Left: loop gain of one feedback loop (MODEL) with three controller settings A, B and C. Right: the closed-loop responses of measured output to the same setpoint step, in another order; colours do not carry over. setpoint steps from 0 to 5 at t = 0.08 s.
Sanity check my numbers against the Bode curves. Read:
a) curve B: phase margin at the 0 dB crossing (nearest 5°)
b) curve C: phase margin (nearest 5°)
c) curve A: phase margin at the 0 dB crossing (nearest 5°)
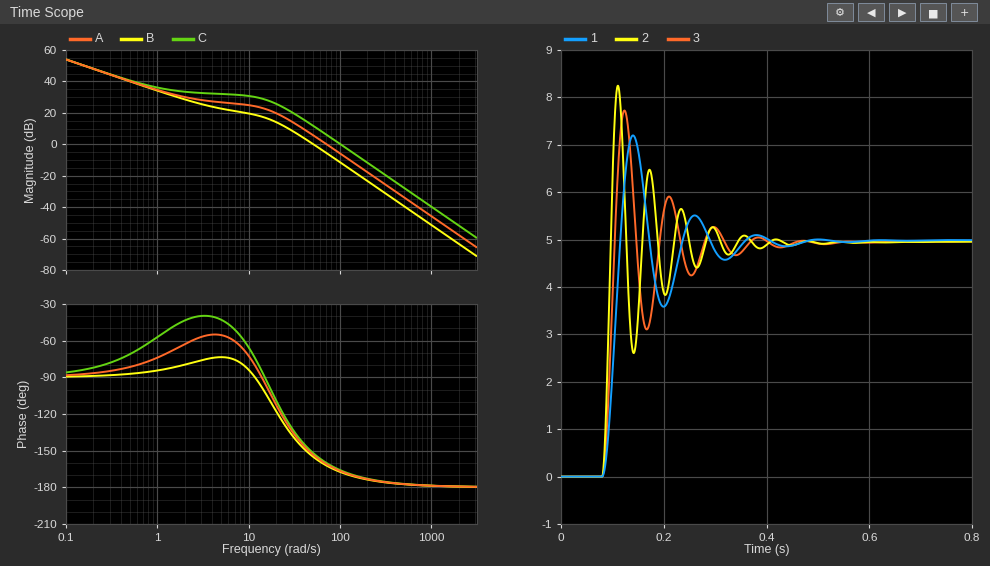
25°
15°
20°
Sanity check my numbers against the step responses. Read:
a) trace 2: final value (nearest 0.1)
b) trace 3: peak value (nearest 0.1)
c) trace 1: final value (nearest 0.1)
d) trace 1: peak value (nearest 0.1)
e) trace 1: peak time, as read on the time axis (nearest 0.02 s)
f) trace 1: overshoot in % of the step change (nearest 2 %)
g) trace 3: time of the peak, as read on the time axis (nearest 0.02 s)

5.0
7.7
5.0
7.2
0.14 s
44 %
0.12 s
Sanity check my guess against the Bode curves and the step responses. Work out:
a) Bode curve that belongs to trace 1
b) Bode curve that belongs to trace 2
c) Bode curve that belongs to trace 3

B
C
A
